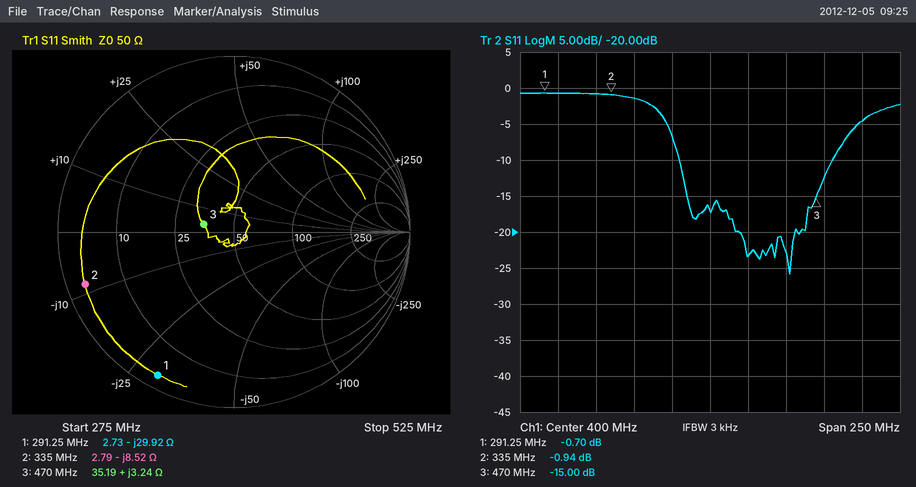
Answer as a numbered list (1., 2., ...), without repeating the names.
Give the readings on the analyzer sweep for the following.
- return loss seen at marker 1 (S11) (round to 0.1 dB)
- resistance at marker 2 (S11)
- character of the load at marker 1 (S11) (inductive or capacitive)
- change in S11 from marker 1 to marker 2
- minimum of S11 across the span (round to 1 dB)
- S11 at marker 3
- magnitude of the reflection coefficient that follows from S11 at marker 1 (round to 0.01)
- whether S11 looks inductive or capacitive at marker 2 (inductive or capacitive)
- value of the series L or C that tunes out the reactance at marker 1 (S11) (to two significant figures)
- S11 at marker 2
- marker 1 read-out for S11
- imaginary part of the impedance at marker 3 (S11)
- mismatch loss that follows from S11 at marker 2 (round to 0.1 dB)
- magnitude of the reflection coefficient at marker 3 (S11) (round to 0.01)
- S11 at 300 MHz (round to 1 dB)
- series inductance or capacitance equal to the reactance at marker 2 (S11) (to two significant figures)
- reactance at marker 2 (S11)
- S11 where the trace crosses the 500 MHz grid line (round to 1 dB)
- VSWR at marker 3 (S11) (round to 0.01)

1. 0.7 dB
2. 2.79 Ω
3. capacitive
4. -0.24 dB
5. -26 dB
6. -15.00 dB
7. 0.92
8. capacitive
9. 16 nH
10. -0.94 dB
11. -0.70 dB
12. +3.24 Ω
13. 7.1 dB
14. 0.18
15. -1 dB
16. 56 pF
17. -8.52 Ω
18. -5 dB
19. 1.43
